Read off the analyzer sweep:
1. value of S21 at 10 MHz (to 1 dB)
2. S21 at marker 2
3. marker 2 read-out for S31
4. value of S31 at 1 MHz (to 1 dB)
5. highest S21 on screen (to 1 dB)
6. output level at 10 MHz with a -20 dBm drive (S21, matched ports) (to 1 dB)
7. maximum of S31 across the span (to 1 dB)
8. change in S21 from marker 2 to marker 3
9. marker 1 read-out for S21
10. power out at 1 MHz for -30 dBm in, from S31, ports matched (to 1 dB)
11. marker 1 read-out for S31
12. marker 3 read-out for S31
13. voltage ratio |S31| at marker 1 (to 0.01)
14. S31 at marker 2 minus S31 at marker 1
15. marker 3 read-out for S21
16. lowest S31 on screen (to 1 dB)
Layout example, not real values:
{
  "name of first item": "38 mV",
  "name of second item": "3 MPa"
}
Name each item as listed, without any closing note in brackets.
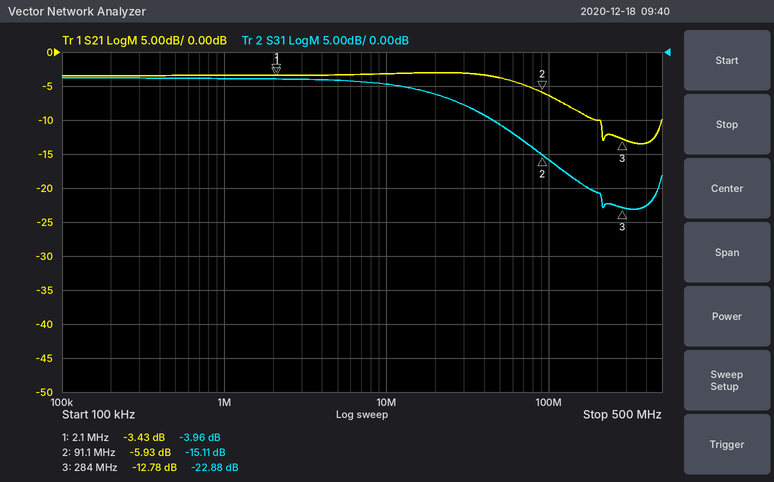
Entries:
{
  "value of S21 at 10 MHz": "-3 dB",
  "S21 at marker 2": "-5.93 dB",
  "marker 2 read-out for S31": "-15.11 dB",
  "value of S31 at 1 MHz": "-4 dB",
  "highest S21 on screen": "-3 dB",
  "output level at 10 MHz with a -20 dBm drive (S21, matched ports)": "-23 dBm",
  "maximum of S31 across the span": "-4 dB",
  "change in S21 from marker 2 to marker 3": "-6.85 dB",
  "marker 1 read-out for S21": "-3.43 dB",
  "power out at 1 MHz for -30 dBm in, from S31, ports matched": "-34 dBm",
  "marker 1 read-out for S31": "-3.96 dB",
  "marker 3 read-out for S31": "-22.88 dB",
  "voltage ratio |S31| at marker 1": "0.63",
  "S31 at marker 2 minus S31 at marker 1": "-11.15 dB",
  "marker 3 read-out for S21": "-12.78 dB",
  "lowest S31 on screen": "-23 dB"
}
